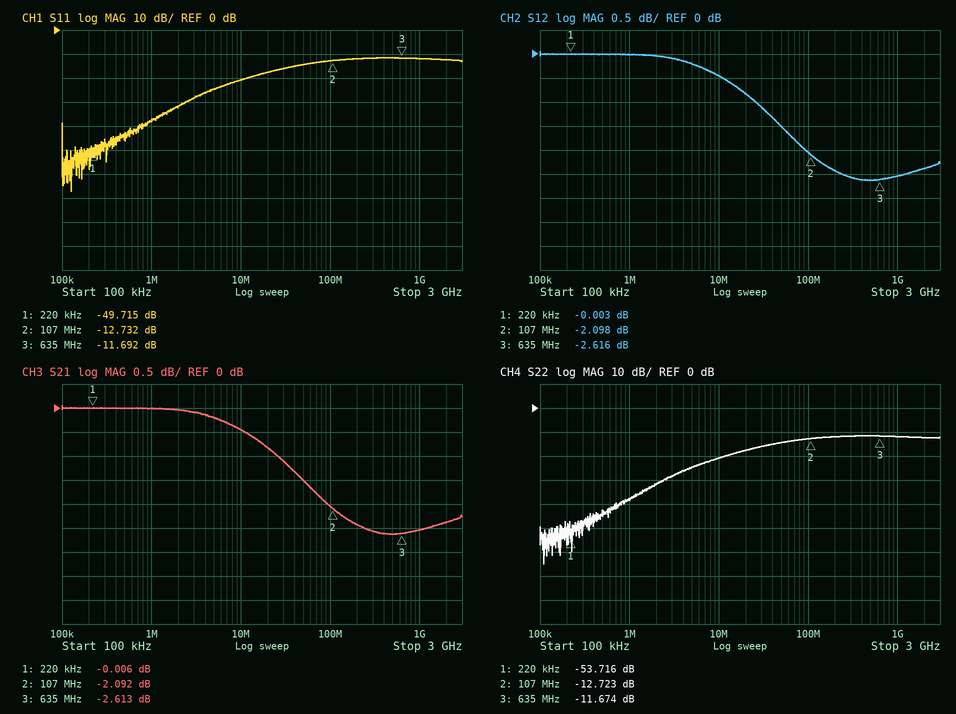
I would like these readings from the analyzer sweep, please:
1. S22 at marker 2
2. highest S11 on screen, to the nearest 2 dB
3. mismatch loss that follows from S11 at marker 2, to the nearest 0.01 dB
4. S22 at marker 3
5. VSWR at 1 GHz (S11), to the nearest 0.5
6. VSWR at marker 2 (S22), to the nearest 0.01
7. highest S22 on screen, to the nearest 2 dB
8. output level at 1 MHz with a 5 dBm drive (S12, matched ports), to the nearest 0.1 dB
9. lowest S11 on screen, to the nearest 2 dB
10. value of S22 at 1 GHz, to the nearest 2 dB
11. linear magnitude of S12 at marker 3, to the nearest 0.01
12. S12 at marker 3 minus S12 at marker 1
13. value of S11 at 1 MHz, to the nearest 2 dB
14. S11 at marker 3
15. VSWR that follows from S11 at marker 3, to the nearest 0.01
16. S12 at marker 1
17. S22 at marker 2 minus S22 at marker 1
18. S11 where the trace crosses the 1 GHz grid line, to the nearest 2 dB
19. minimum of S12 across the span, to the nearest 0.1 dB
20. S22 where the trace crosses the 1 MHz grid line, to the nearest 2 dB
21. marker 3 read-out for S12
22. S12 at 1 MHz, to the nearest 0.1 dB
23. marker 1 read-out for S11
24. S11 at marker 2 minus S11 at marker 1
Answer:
-12.723 dB
-12 dB
0.24 dB
-11.674 dB
1.5
1.60
-12 dB
5.0 dBm
-68 dB
-12 dB
0.74
-2.613 dB
-38 dB
-11.692 dB
1.70
-0.003 dB
40.993 dB
-12 dB
-2.6 dB
-38 dB
-2.616 dB
0.0 dB
-49.715 dB
36.983 dB
